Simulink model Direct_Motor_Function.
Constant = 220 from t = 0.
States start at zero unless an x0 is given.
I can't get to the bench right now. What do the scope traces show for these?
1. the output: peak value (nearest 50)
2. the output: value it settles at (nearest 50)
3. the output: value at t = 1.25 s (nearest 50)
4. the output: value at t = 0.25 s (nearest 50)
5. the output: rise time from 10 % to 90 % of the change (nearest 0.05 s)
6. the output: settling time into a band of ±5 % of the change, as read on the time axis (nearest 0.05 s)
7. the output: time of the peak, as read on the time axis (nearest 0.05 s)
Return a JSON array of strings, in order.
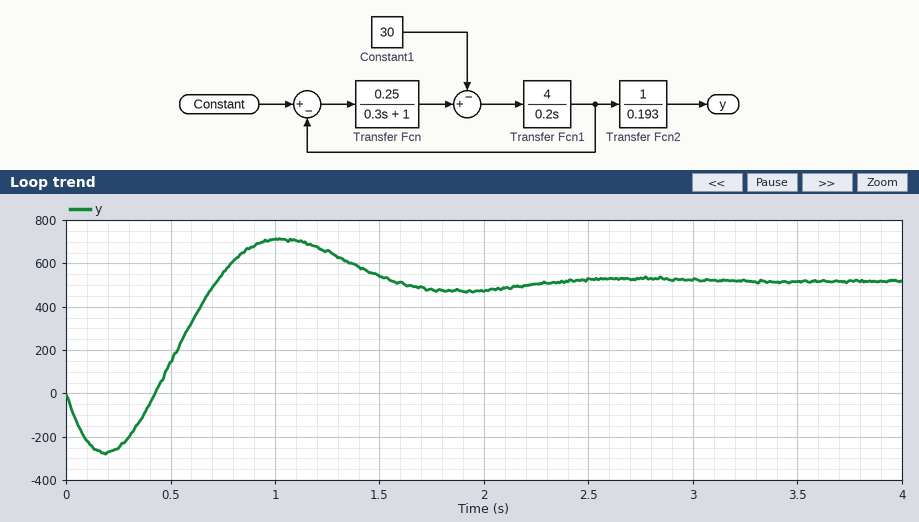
["700", "500", "650", "-250", "0.25 s", "2.15 s", "1.05 s"]
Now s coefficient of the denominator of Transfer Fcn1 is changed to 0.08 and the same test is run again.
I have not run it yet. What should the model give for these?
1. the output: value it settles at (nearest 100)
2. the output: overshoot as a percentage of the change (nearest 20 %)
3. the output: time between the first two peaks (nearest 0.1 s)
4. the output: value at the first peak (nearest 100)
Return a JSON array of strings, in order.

["500", "100 %", "1.0 s", "1000"]
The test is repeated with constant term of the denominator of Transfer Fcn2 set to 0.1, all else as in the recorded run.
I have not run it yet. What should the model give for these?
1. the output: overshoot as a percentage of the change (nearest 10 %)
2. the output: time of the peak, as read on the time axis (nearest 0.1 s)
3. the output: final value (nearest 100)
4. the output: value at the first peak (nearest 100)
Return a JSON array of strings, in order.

["40 %", "1.0 s", "1000", "1400"]
